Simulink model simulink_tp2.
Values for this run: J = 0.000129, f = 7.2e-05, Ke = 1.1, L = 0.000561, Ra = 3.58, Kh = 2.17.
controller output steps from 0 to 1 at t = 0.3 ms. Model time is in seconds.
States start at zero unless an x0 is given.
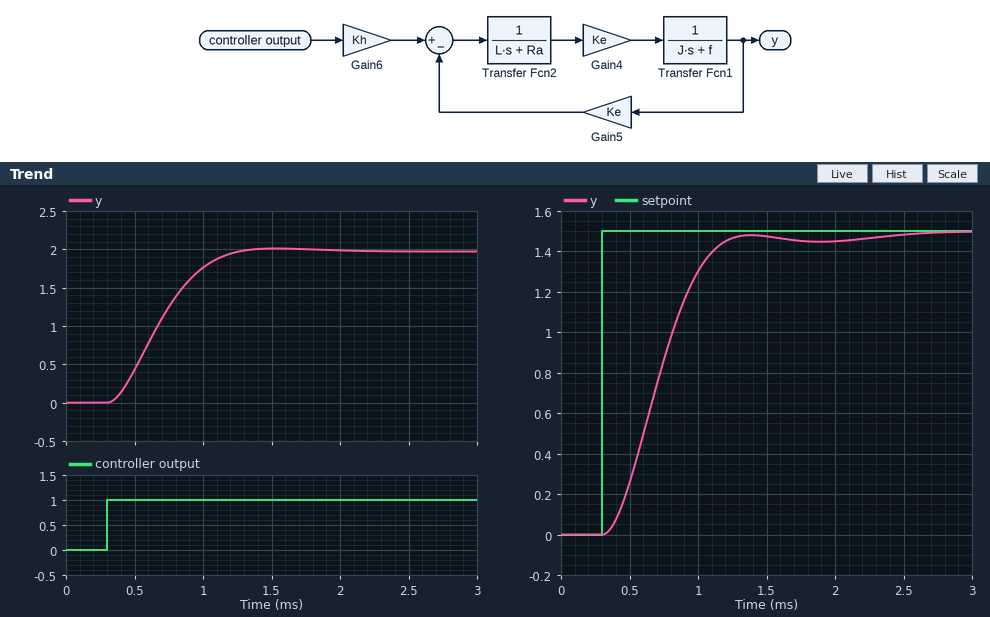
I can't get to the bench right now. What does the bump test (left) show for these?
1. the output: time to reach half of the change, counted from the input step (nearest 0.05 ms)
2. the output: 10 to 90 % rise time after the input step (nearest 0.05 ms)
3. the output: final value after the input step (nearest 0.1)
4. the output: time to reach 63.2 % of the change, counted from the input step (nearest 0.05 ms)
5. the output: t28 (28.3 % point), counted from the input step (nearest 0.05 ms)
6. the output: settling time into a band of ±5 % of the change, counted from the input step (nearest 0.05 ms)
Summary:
0.35 ms
0.60 ms
2.0
0.45 ms
0.25 ms
0.80 ms
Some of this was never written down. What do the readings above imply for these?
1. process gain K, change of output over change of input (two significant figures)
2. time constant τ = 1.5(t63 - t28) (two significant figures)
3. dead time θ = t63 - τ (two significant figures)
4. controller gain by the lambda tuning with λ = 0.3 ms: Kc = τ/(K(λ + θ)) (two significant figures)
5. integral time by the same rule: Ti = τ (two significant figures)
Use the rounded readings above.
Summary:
2.0
0.30 ms
0.15 ms
0.33
0.30 ms
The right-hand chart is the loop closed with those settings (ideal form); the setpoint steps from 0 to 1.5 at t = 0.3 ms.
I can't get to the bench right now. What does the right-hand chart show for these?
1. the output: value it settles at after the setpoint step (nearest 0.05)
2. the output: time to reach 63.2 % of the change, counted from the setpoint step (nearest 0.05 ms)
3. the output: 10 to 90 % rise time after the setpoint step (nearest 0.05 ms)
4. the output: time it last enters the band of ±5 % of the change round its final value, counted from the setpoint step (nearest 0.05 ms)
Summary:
1.50
0.50 ms
0.60 ms
0.85 ms
